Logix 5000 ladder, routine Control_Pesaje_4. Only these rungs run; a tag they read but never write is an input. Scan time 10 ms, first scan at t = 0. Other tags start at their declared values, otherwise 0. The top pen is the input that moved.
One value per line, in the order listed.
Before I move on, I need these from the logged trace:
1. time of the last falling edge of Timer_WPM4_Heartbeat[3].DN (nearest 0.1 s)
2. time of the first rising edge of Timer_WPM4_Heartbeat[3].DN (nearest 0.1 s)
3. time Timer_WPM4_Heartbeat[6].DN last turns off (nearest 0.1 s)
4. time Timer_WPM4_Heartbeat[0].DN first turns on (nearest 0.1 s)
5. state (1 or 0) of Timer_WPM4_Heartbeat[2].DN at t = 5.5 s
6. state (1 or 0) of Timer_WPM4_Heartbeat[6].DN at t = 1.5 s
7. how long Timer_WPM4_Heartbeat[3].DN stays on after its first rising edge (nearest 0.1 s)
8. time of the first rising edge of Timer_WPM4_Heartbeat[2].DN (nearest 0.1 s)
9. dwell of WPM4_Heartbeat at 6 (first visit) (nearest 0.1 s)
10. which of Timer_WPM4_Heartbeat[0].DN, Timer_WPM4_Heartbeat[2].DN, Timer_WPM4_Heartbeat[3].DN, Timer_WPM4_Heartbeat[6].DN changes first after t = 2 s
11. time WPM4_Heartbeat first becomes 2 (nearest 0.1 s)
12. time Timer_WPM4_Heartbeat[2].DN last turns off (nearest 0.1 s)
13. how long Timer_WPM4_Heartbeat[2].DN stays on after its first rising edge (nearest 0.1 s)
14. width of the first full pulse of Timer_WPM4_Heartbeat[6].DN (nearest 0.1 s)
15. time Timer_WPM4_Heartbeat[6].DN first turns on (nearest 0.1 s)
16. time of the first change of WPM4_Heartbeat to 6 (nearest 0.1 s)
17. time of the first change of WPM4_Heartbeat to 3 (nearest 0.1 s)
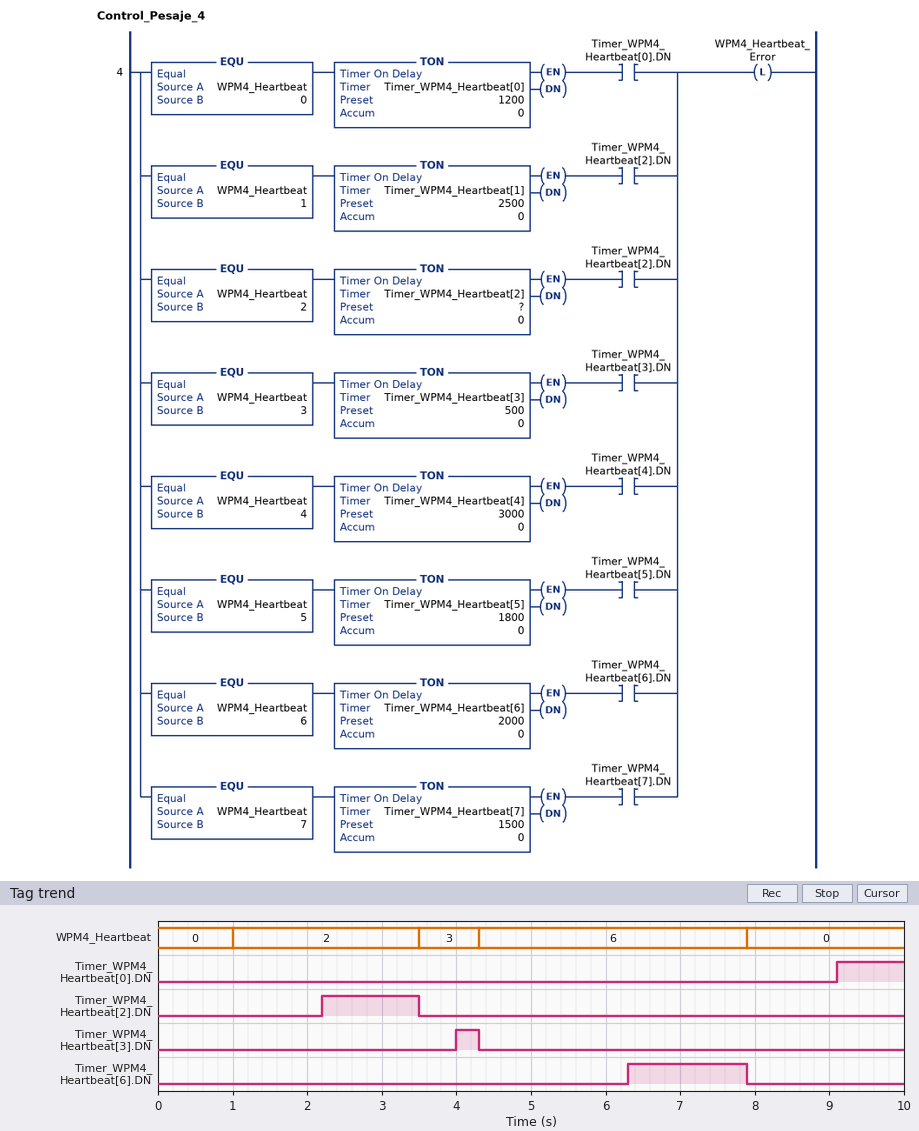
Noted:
4.3 s
4.0 s
7.9 s
9.1 s
0
0
0.3 s
2.2 s
3.6 s
Timer_WPM4_Heartbeat[2].DN
1.0 s
3.5 s
1.3 s
1.6 s
6.3 s
4.3 s
3.5 s
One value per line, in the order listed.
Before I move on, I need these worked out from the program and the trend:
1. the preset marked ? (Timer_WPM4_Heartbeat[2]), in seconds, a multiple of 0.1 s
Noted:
1.2 s
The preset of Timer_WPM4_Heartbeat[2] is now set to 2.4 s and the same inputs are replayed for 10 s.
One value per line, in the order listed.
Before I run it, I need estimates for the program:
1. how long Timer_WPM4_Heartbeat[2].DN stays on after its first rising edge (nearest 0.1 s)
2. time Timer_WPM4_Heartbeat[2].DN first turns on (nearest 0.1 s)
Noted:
0.1 s
3.4 s
